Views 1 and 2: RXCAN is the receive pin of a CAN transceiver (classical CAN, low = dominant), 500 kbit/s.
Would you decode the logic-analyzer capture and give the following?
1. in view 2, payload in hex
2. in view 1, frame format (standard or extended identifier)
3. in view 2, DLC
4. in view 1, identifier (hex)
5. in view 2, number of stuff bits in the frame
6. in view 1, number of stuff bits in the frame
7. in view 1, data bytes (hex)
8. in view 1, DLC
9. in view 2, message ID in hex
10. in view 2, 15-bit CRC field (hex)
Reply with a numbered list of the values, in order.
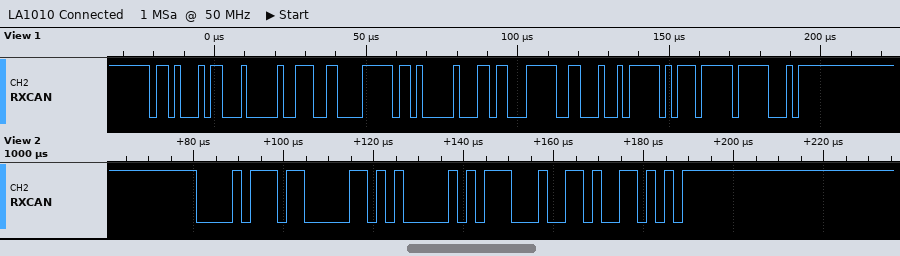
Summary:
1. A0 5C
2. standard
3. 2
4. 0x68B
5. 2
6. 7
7. 0E 61 FD 00 D8 FB 12 FD
8. 8
9. 0x0BB
10. 0x269A
